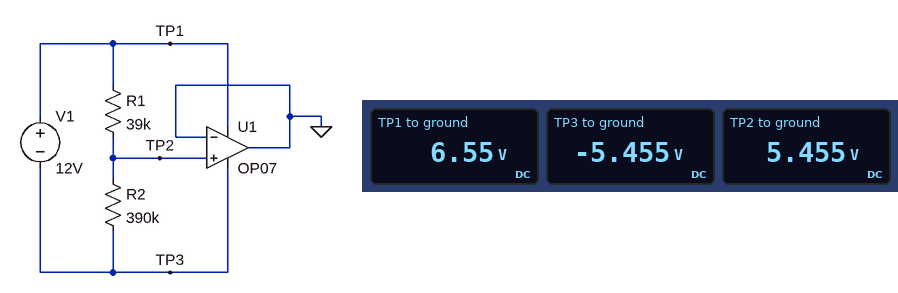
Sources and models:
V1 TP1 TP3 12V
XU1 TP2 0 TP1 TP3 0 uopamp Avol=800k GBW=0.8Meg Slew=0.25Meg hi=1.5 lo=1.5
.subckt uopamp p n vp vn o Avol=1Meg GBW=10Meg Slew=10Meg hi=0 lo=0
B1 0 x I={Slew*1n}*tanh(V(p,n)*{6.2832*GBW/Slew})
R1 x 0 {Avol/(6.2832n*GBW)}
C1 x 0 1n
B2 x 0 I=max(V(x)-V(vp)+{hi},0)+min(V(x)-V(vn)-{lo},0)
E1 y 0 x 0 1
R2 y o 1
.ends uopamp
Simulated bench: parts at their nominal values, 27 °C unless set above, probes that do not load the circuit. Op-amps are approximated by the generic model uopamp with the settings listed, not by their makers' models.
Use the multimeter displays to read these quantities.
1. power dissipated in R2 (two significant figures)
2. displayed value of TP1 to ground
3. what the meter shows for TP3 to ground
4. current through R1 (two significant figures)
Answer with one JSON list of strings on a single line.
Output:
["310 µW", "6.55 V", "-5.455 V", "28 µA"]
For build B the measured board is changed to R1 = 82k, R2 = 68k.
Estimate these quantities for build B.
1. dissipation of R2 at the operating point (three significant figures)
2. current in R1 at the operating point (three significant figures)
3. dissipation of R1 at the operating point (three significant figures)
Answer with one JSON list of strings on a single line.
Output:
["435 µW", "80.0 µA", "525 µW"]
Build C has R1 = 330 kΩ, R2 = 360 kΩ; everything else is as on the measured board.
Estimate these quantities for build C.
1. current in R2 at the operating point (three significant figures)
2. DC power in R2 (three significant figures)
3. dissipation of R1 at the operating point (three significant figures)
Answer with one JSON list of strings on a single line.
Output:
["17.4 µA", "109 µW", "99.8 µW"]
